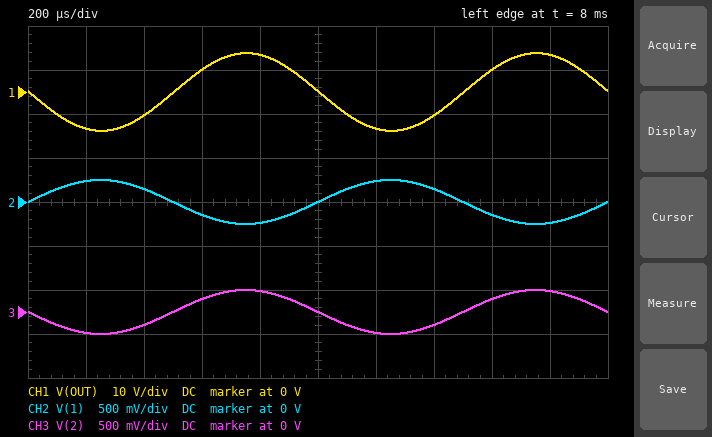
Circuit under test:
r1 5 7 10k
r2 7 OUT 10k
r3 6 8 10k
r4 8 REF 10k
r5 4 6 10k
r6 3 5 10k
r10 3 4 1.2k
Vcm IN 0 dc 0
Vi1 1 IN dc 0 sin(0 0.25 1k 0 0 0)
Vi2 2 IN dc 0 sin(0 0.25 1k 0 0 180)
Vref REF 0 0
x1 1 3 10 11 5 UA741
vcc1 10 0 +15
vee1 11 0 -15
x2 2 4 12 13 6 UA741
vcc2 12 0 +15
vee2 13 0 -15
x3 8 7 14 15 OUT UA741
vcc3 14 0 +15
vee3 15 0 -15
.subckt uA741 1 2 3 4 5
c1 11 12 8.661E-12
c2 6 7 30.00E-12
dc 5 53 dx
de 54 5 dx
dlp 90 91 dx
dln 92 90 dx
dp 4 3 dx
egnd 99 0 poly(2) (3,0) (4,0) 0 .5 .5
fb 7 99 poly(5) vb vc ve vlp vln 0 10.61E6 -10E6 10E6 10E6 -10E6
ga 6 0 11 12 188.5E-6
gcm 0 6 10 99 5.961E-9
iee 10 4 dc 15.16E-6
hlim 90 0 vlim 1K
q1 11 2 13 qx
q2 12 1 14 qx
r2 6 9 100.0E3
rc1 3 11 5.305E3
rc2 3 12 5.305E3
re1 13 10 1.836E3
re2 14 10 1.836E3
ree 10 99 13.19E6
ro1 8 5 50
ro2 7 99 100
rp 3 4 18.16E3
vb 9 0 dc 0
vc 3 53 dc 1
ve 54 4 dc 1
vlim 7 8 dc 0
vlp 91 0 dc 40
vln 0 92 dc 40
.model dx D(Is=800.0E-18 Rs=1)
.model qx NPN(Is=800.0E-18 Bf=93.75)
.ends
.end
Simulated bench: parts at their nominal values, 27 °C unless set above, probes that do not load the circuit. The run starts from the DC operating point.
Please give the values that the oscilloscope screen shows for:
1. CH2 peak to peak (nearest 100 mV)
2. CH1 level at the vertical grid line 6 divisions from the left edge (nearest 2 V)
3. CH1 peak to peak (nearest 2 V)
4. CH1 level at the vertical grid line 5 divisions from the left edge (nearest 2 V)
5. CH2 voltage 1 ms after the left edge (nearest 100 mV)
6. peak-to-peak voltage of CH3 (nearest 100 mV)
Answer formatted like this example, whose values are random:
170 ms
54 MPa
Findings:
500 mV
-8 V
18 V
0 V
0 V
500 mV
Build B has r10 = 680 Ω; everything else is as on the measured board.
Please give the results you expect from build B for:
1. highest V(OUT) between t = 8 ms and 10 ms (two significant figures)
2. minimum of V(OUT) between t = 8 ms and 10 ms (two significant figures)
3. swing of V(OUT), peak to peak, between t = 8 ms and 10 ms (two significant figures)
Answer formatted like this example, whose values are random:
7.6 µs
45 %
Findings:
15 V
-15 V
29 V
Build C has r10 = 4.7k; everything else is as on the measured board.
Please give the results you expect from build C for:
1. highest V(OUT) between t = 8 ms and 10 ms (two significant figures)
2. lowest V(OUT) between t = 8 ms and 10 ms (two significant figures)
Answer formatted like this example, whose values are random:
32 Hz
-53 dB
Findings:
2.6 V
-2.6 V
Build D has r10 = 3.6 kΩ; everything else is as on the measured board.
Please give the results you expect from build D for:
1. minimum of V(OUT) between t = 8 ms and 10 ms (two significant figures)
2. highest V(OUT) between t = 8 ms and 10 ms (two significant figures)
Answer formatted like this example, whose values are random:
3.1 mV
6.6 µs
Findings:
-3.3 V
3.3 V
